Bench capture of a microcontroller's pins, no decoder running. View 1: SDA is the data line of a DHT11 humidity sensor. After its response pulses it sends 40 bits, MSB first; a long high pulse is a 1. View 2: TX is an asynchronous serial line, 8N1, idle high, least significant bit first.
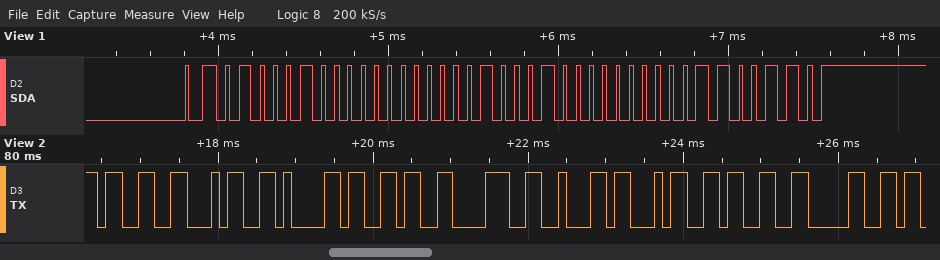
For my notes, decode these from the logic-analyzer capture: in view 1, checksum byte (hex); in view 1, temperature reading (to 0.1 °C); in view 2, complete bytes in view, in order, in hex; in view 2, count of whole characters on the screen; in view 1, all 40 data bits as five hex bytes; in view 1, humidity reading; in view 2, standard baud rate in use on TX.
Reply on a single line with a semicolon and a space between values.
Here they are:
0x66; 34.0 °C; 33 34 61 36 38 62 34 33 30; 9; 44 00 22 00 66; 68 %; 9600 baud
